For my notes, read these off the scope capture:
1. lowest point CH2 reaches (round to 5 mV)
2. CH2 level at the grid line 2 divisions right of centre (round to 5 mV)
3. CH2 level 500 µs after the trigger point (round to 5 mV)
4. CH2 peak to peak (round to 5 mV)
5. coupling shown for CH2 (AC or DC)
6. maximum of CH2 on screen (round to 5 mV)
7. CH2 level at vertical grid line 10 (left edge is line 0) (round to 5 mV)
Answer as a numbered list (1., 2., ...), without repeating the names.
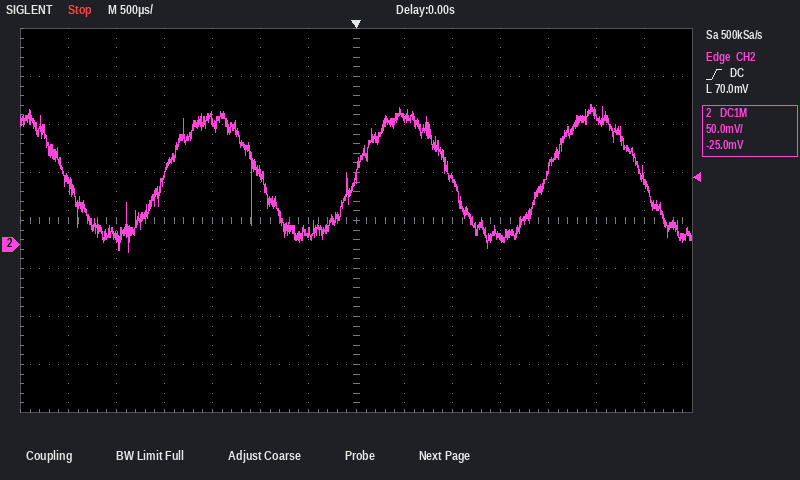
1. -10 mV
2. 70 mV
3. 130 mV
4. 155 mV
5. DC
6. 145 mV
7. 5 mV
